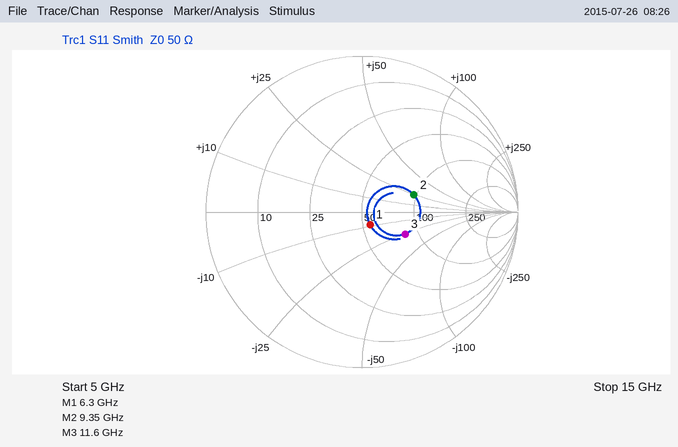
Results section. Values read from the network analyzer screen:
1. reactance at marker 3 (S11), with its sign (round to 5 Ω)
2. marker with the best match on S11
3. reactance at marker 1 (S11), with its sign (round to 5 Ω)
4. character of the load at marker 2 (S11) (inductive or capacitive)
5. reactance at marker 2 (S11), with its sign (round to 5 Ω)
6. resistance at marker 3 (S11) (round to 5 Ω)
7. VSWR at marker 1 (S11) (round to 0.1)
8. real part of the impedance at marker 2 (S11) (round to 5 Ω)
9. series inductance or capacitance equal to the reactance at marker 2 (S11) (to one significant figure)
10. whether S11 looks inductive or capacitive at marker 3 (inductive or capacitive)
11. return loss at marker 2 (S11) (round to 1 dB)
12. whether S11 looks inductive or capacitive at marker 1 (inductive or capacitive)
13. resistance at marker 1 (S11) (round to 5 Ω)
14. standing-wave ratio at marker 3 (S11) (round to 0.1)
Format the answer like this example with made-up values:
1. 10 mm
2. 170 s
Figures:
1. -25 Ω
2. marker 1
3. -10 Ω
4. inductive
5. +25 Ω
6. 85 Ω
7. 1.2
8. 95 Ω
9. 400 pH
10. capacitive
11. 9 dB
12. capacitive
13. 55 Ω
14. 1.9
